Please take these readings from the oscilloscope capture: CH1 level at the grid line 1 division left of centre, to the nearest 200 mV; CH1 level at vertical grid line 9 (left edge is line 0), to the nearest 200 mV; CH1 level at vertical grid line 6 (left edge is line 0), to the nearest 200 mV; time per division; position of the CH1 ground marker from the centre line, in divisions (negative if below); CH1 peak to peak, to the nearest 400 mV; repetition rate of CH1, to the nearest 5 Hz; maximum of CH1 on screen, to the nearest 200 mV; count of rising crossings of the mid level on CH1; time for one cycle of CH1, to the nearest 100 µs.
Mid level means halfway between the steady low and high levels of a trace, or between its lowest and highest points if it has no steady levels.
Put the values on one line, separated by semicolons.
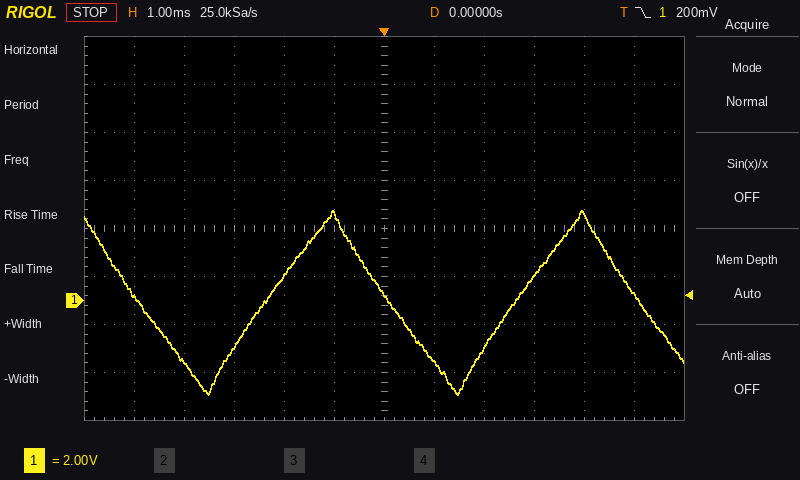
3.6 V; 1.0 V; 200 mV; 1 ms; -1.5 div; 7.6 V; 200 Hz; 3.8 V; 2; 5.0 ms
